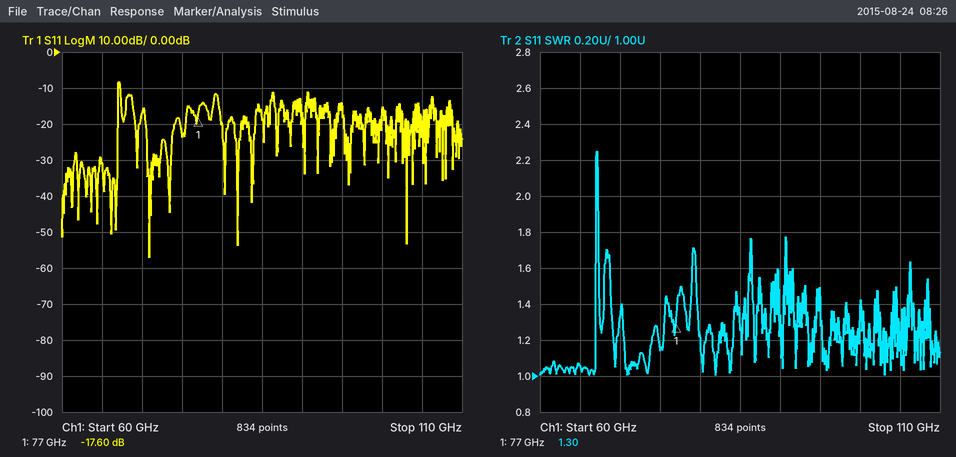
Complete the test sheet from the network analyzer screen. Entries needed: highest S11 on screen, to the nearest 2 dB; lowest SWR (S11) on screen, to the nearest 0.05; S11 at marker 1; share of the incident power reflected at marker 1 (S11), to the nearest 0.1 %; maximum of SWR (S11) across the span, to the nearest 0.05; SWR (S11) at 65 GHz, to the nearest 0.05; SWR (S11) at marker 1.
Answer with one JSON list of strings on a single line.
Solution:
["-8 dB", "1.00", "-17.60 dB", "1.7 %", "2.25", "1.05", "1.30"]
